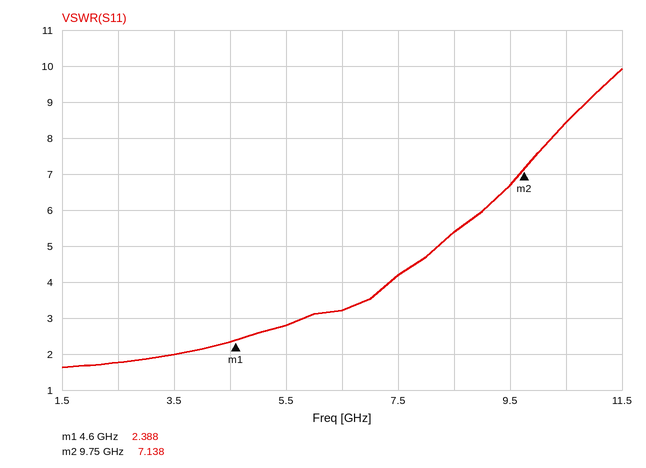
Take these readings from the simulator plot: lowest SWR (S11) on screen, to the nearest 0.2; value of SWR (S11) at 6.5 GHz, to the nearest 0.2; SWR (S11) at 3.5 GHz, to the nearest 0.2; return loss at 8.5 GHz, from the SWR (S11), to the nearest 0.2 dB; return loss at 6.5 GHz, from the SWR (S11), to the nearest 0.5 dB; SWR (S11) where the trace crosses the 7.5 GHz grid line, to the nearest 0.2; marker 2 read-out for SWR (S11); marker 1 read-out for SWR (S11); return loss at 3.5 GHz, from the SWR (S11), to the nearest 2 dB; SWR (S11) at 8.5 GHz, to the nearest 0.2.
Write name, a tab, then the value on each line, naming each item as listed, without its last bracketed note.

lowest SWR (S11) on screen, to the nearest 0.2	1.6
value of SWR (S11) at 6.5 GHz, to the nearest 0.2	3.2
SWR (S11) at 3.5 GHz, to the nearest 0.2	2.0
return loss at 8.5 GHz, from the SWR (S11), to the nearest 0.2 dB	3.2 dB
return loss at 6.5 GHz, from the SWR (S11), to the nearest 0.5 dB	5.5 dB
SWR (S11) where the trace crosses the 7.5 GHz grid line, to the nearest 0.2	4.2
marker 2 read-out for SWR	7.138
marker 1 read-out for SWR	2.388
return loss at 3.5 GHz, from the SWR (S11), to the nearest 2 dB	10 dB
SWR (S11) at 8.5 GHz, to the nearest 0.2	5.4
